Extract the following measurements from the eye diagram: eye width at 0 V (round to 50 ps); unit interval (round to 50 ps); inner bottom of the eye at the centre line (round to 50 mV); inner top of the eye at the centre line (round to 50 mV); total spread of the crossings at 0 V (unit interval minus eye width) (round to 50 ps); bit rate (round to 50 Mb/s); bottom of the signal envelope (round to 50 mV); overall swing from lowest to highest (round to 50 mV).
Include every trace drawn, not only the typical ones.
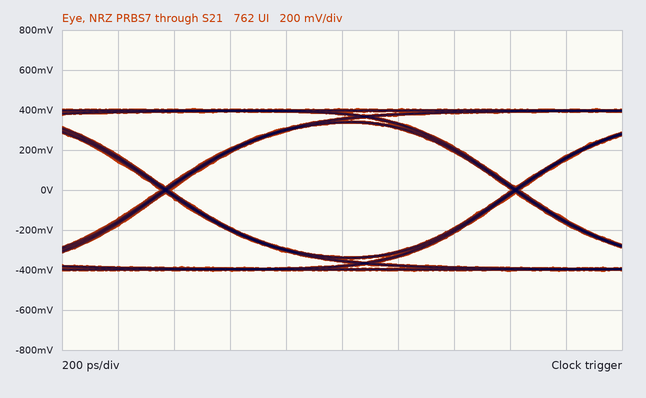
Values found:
1.20 ns
1.25 ns
-350 mV
350 mV
50 ps
800 Mb/s
-400 mV
800 mV
